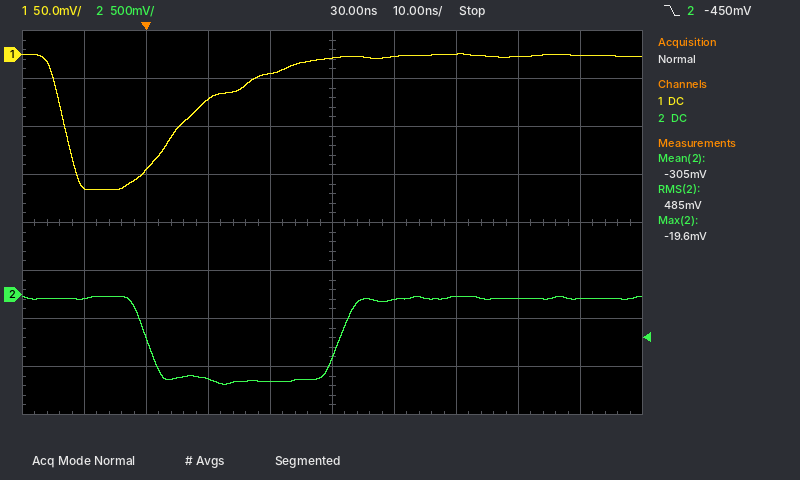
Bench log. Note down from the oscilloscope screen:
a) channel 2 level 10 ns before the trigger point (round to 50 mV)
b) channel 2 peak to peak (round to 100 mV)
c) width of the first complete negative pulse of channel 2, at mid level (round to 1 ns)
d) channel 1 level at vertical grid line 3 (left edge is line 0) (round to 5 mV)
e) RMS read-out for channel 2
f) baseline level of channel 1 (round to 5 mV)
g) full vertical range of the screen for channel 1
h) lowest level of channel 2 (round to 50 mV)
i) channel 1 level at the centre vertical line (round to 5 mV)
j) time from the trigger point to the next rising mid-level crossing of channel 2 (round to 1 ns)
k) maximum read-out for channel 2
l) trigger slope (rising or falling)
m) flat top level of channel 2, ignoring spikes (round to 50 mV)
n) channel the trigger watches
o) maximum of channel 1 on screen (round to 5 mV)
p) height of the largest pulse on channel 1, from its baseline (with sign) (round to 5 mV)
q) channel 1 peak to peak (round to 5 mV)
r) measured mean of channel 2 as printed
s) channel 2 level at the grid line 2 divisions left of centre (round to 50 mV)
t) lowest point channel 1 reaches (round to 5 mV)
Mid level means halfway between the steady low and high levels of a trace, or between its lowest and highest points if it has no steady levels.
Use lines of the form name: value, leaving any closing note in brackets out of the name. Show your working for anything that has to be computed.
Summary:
channel 2 level 10 ns before the trigger point: -50 mV
channel 2 peak to peak: 900 mV
width of the first complete negative pulse of channel 2, at mid level: 31 ns
channel 1 level at vertical grid line 3 (left edge is line 0): -45 mV
RMS read-out for channel 2: 485 mV
baseline level of channel 1: 0 mV
full vertical range of the screen for channel 1: 400 mV
lowest level of channel 2: -950 mV
channel 1 level at the centre vertical line: -5 mV
time from the trigger point to the next rising mid-level crossing of channel 2: 31 ns
maximum read-out for channel 2: -19.6 mV
trigger slope: falling
flat top level of channel 2, ignoring spikes: -50 mV
channel the trigger watches: channel 2
maximum of channel 1 on screen: 0 mV
height of the largest pulse on channel 1, from its baseline (with sign): -140 mV − (0 mV) = -140 mV
channel 1 peak to peak: 0 mV − (-140 mV) = 140 mV
measured mean of channel 2 as printed: -305 mV
channel 2 level at the grid line 2 divisions left of centre: -900 mV
lowest point channel 1 reaches: -140 mV
